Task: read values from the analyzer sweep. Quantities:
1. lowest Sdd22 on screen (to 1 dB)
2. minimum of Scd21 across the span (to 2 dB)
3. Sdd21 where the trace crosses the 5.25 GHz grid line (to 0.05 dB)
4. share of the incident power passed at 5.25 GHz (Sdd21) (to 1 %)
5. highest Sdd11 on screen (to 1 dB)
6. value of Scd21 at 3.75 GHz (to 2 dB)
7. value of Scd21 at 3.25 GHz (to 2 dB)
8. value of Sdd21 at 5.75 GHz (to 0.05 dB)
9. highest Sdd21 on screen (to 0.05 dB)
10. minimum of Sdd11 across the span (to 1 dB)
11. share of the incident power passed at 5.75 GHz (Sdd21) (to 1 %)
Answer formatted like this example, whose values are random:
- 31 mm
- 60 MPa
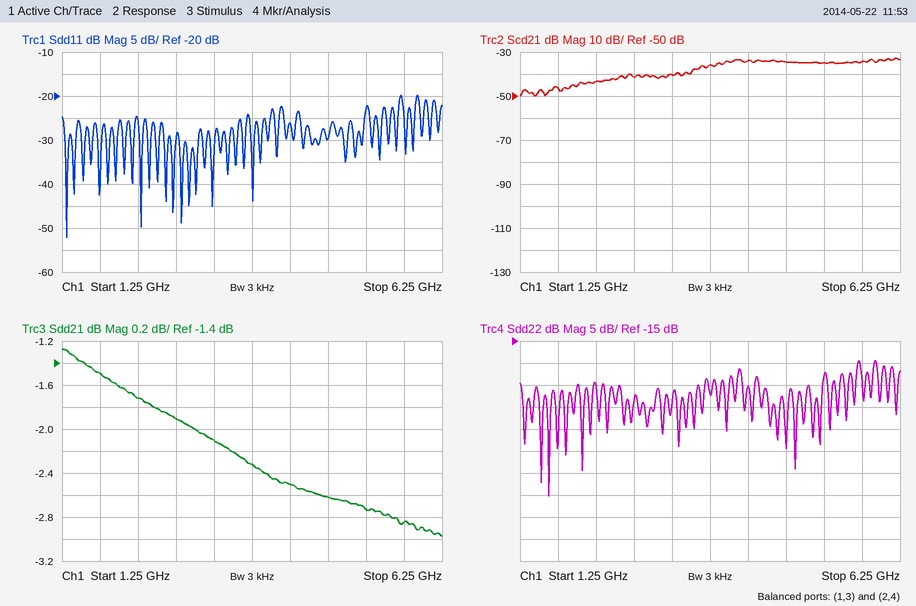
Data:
- -50 dB
- -50 dB
- -2.75 dB
- 53 %
- -20 dB
- -36 dB
- -40 dB
- -2.85 dB
- -1.25 dB
- -52 dB
- 52 %
